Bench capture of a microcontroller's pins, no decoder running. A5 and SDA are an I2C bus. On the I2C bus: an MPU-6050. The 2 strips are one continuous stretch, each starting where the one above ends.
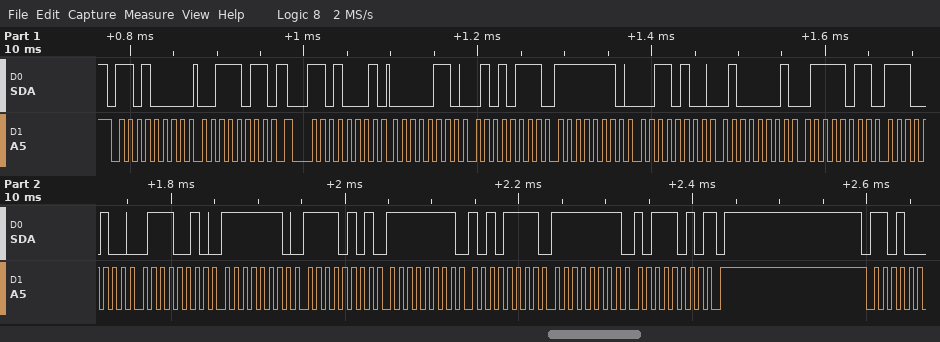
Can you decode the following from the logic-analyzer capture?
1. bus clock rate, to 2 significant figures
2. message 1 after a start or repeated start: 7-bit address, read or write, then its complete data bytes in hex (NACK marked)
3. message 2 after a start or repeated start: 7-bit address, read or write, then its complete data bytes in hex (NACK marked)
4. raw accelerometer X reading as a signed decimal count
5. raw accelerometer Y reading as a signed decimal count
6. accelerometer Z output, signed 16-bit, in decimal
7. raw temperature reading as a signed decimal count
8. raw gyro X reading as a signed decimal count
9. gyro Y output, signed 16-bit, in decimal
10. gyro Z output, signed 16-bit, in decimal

100 kHz
0x68 write: 3B
0x68 read: 06 57 FE 34 41 7B E4 72 FE F5 FF AF FF BA NACK
1623
-460
16763
-7054
-267
-81
-70
